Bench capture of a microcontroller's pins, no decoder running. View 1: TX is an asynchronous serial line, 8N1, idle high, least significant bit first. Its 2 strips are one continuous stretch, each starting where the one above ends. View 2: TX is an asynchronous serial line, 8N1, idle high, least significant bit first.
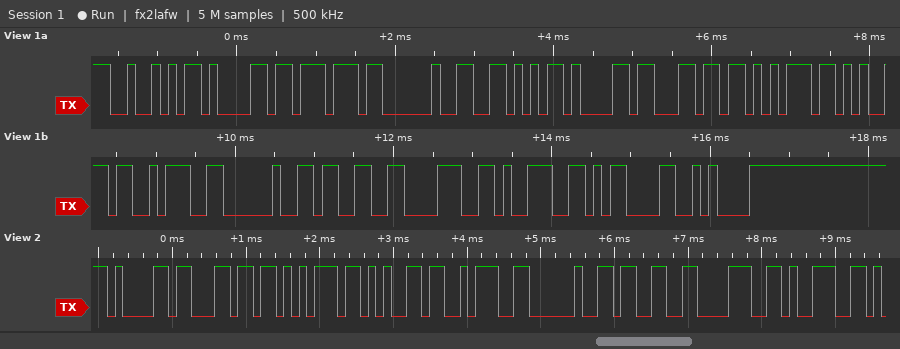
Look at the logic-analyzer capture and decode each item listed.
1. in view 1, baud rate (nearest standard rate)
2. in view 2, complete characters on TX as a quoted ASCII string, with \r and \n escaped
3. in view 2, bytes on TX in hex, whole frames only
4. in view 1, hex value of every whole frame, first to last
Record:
9600 baud
"alue: 389"
61 6C 75 65 3A 20 33 38 39
52 61 77 20 56 61 6C 75 65 3A 20 33 38 39 0D 0A
